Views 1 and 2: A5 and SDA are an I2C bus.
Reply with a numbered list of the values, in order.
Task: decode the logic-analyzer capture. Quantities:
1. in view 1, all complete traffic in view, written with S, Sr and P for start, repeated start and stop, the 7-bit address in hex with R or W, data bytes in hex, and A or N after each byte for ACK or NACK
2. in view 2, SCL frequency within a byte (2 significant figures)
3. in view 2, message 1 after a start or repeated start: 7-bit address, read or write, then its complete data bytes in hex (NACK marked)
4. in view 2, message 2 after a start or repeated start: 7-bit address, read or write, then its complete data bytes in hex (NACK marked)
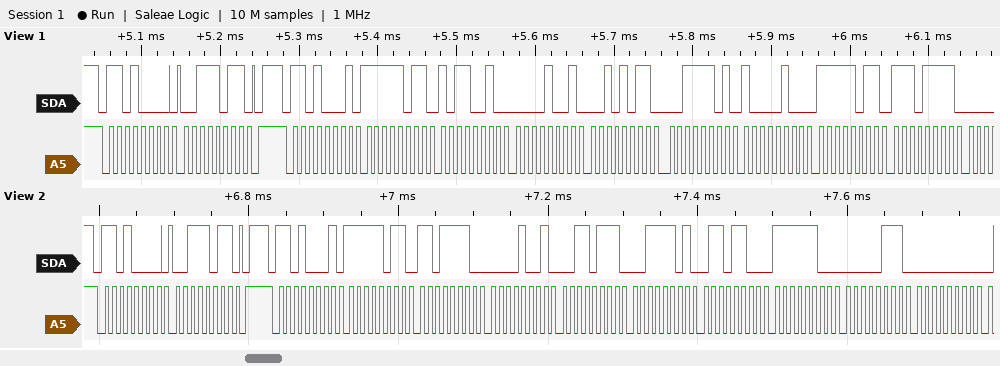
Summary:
1. S 68W A 3B A P S 68R A FB A B2 A 09 A 2B A 3D A 84 A FB A EF A
2. 100 kHz
3. 0x68 write: 3B
4. 0x68 read: FB DE 09 37 3D 6C FC 07 00
